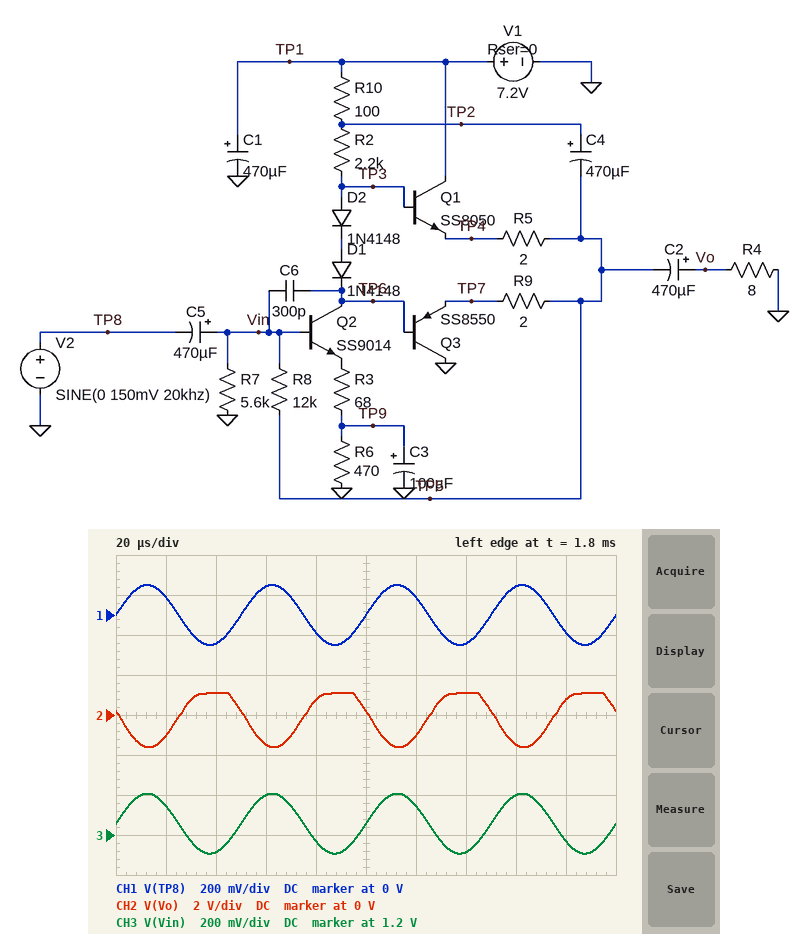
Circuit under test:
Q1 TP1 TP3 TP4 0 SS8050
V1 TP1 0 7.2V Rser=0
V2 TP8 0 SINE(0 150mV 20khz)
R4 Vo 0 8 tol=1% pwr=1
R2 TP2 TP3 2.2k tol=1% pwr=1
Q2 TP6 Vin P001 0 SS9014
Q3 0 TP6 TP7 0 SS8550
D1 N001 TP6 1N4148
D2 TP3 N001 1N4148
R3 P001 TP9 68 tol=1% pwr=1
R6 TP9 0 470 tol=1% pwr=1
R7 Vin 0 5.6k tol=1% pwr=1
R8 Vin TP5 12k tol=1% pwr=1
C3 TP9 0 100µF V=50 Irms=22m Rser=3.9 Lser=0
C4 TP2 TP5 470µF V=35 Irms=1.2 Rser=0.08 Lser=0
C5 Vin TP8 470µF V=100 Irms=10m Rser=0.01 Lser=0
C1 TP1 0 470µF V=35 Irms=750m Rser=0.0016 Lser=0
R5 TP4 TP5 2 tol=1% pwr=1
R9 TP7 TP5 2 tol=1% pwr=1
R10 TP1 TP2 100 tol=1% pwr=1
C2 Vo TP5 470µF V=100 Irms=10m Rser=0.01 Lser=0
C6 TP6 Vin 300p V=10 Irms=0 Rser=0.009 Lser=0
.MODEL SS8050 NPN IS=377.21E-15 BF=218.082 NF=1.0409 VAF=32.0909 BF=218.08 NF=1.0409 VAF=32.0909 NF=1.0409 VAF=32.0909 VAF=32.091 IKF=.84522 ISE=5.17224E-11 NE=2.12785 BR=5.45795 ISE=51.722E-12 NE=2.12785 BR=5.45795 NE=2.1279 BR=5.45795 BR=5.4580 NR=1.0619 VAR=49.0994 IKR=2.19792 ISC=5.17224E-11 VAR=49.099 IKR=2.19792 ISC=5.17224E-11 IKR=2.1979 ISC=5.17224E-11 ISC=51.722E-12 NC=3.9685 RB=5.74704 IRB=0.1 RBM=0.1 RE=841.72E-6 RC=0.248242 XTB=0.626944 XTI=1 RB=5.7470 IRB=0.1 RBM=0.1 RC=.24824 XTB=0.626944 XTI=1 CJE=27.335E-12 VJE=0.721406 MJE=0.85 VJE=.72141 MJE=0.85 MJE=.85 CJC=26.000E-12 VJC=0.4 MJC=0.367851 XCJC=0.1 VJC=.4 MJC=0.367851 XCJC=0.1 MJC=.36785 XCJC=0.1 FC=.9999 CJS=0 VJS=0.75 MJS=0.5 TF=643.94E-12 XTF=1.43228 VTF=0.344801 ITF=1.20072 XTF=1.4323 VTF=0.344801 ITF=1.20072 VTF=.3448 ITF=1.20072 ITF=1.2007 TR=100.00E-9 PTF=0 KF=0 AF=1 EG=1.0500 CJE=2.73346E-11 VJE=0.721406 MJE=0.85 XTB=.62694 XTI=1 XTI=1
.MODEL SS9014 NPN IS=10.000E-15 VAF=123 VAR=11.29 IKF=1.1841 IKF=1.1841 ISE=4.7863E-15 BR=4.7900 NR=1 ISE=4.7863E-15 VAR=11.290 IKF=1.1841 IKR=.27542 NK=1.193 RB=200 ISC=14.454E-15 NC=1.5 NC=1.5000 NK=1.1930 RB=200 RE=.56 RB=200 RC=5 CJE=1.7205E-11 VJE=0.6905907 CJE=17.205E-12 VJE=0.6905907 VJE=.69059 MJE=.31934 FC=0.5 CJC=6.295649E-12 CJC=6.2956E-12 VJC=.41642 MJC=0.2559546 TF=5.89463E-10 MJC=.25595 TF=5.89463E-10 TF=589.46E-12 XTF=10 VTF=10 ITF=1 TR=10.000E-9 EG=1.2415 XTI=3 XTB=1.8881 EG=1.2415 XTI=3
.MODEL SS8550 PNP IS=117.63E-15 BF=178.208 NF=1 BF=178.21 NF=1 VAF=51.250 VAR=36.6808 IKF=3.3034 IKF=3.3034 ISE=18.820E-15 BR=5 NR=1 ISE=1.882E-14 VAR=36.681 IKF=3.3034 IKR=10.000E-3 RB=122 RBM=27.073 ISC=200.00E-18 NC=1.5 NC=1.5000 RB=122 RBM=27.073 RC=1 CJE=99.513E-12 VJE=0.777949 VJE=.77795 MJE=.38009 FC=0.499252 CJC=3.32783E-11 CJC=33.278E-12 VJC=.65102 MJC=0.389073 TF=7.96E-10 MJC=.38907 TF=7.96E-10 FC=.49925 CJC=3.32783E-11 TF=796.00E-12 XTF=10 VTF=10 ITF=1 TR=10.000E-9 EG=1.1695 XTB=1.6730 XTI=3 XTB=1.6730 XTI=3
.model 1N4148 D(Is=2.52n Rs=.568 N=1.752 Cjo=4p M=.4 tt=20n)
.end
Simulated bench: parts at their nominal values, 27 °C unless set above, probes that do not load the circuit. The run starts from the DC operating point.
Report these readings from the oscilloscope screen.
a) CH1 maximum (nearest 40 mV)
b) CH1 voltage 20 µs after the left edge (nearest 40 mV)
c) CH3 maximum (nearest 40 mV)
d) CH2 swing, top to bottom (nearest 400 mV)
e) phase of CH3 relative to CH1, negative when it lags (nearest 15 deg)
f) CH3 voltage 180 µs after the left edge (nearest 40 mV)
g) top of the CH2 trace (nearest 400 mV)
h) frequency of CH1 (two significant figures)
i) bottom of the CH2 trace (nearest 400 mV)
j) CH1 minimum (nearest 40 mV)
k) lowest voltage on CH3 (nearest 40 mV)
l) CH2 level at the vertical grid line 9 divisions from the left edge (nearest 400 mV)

160 mV
80 mV
1.40 V
2.8 V
0 deg
1.16 V
1.2 V
20 kHz
-1.6 V
-160 mV
1.12 V
800 mV
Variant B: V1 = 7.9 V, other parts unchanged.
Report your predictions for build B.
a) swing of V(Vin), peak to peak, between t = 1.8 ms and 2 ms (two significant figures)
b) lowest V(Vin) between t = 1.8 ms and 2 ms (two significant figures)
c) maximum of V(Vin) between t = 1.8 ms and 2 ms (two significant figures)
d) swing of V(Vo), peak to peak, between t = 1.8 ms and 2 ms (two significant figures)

300 mV
1.2 V
1.5 V
2.8 V
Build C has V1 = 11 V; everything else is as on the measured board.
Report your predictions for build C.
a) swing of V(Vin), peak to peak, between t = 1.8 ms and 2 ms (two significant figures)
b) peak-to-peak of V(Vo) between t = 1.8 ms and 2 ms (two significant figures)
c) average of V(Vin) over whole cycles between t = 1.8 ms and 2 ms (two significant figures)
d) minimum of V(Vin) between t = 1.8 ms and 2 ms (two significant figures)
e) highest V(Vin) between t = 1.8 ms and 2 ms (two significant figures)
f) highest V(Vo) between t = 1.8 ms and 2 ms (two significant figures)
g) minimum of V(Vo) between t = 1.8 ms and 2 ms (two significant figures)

300 mV
3.0 V
1.8 V
1.6 V
1.9 V
1.2 V
-1.8 V
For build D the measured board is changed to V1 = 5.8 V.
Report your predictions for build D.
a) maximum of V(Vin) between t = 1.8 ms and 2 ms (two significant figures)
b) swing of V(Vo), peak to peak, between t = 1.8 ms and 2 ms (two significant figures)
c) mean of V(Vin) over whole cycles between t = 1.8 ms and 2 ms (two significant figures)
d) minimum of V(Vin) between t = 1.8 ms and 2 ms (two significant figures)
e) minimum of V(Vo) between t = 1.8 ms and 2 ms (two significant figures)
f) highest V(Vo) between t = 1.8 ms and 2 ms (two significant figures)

1.2 V
2.3 V
1.1 V
920 mV
-1.5 V
820 mV
